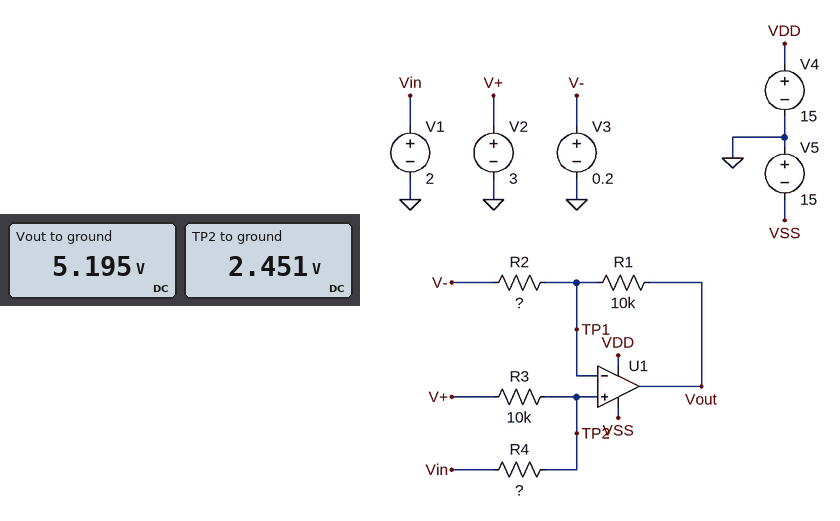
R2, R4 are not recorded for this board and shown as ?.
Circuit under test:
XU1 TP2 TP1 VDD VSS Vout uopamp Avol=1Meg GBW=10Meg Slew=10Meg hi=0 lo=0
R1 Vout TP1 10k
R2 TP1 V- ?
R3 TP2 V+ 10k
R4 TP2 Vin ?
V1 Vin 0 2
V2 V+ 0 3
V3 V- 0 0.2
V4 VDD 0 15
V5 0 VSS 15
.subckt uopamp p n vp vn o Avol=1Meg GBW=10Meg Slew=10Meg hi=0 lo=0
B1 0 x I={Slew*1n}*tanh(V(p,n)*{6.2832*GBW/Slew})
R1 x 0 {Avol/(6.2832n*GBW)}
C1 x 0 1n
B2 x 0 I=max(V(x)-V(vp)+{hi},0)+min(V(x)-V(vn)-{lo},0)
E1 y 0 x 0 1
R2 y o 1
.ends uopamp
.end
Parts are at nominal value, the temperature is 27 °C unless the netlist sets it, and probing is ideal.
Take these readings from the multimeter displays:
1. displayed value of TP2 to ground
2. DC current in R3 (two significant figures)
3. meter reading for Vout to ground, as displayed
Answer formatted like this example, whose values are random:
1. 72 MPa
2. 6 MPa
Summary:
1. 2.451 V
2. 55 µA
3. 5.195 V
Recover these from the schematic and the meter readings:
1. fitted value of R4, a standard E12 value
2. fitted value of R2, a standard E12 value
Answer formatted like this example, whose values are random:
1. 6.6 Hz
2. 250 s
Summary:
1. 8.2 kΩ
2. 8.2 kΩ
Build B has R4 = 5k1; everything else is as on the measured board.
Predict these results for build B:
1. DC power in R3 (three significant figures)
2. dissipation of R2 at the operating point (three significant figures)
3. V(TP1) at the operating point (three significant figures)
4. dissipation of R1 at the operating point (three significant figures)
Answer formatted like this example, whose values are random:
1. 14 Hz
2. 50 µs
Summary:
1. 43.9 µW
2. 557 µW
3. 2.34 V
4. 680 µW
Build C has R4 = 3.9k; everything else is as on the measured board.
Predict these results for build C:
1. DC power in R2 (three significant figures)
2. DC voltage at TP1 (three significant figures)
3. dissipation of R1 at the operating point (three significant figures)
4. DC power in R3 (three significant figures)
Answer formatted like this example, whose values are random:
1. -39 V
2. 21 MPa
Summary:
1. 528 µW
2. 2.28 V
3. 644 µW
4. 51.8 µW
